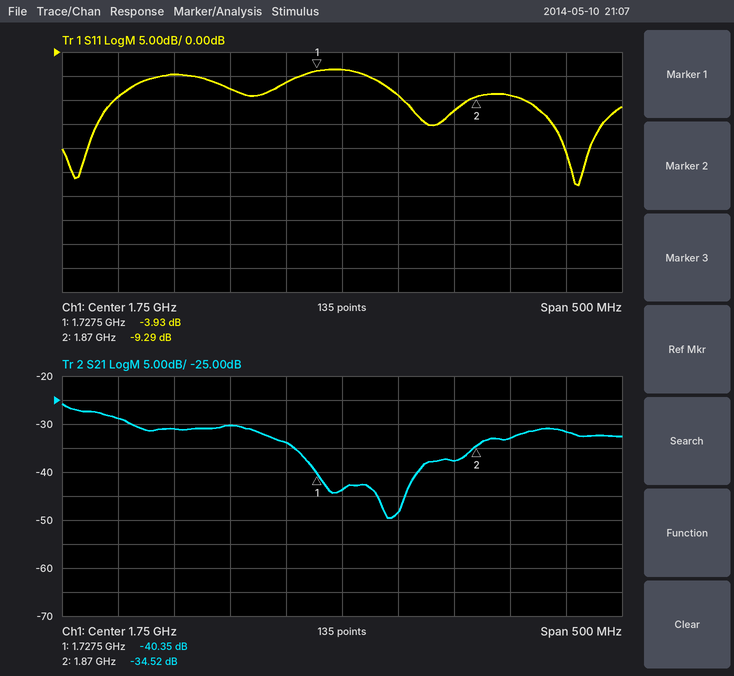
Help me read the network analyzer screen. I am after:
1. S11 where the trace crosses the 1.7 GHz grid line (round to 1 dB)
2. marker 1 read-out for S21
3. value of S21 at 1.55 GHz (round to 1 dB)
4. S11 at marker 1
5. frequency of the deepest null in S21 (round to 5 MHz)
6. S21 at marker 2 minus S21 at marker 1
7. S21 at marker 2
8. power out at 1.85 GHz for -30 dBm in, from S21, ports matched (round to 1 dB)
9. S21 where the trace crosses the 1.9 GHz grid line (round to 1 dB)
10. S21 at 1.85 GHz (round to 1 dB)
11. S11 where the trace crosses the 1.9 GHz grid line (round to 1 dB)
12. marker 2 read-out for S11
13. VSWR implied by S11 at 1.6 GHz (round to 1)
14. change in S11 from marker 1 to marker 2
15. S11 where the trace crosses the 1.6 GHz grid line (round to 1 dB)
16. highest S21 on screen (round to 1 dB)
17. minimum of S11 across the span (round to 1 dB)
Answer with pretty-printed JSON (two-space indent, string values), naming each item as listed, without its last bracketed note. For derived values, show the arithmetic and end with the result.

{
  "S11 where the trace crosses the 1.7 GHz grid line": "-6 dB",
  "marker 1 read-out for S21": "-40.35 dB",
  "value of S21 at 1.55 GHz": "-29 dB",
  "S11 at marker 1": "-3.93 dB",
  "frequency of the deepest null in S21": "1.790 GHz",
  "S21 at marker 2 minus S21 at marker 1": "-34.52 − (-40.35) = 5.83 dB",
  "S21 at marker 2": "-34.52 dB",
  "power out at 1.85 GHz for -30 dBm in, from S21, ports matched": "-30 dBm + (-38 dB) = -68 dBm",
  "S21 where the trace crosses the 1.9 GHz grid line": "-33 dB",
  "S21 at 1.85 GHz": "-38 dB",
  "S11 where the trace crosses the 1.9 GHz grid line": "-9 dB",
  "marker 2 read-out for S11": "-9.29 dB",
  "VSWR implied by S11 at 1.6 GHz": "|Γ| = 10^(-5/20) = 0.5623; VSWR = (1 + 0.5623)/(1 − 0.5623) ≈ 4",
  "change in S11 from marker 1 to marker 2": "-9.29 − (-3.93) = -5.36 dB",
  "S11 where the trace crosses the 1.6 GHz grid line": "-5 dB",
  "highest S21 on screen": "-26 dB",
  "minimum of S11 across the span": "-28 dB"
}
